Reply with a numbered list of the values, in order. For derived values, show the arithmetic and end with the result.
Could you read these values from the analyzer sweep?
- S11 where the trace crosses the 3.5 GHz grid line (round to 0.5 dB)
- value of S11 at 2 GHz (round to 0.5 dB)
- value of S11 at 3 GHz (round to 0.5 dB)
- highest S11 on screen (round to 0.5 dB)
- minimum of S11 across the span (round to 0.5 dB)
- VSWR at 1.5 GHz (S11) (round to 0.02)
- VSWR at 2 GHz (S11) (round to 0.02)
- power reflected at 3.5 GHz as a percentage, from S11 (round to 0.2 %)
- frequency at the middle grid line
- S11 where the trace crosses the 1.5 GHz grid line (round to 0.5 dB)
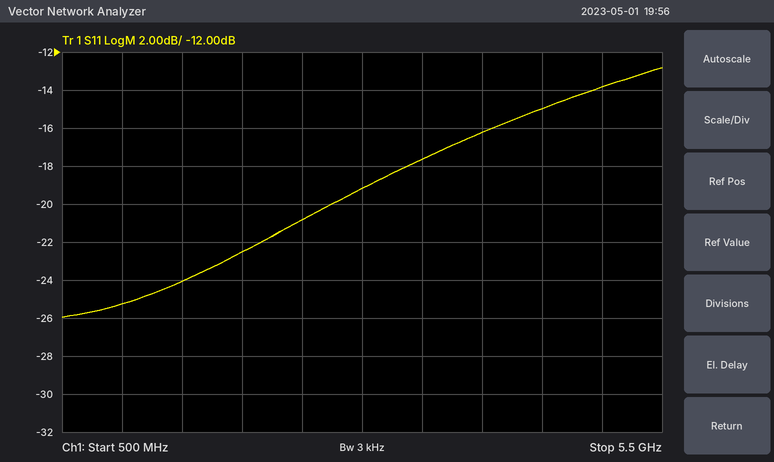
1. -17.5 dB
2. -22.5 dB
3. -19.0 dB
4. -13.0 dB
5. -26.0 dB
6. |Γ| = 10^(-24/20) = 0.0631; VSWR = (1 + 0.0631)/(1 − 0.0631) ≈ 1.13, so 1.14 to the nearest 0.02
7. |Γ| = 10^(-22.5/20) = 0.0750; VSWR = (1 + 0.0750)/(1 − 0.0750) ≈ 1.16
8. 10^(-17.5/10) ≈ 1.8 %
9. 3 GHz
10. -24.0 dB
